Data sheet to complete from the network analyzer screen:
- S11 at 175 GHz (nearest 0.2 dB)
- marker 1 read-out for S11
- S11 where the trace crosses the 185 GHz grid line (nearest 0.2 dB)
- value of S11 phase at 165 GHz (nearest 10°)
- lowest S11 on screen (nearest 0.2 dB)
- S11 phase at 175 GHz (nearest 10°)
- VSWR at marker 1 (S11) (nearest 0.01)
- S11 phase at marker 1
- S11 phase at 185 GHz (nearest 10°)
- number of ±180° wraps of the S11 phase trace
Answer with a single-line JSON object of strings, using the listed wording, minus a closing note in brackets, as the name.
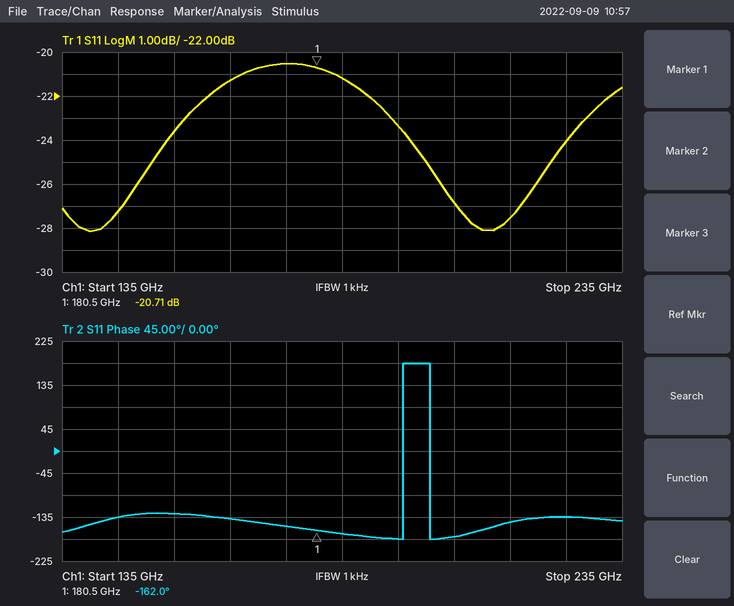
{"S11 at 175 GHz": "-20.6 dB", "marker 1 read-out for S11": "-20.71 dB", "S11 where the trace crosses the 185 GHz grid line": "-21.2 dB", "value of S11 phase at 165 GHz": "-140°", "lowest S11 on screen": "-28.2 dB", "S11 phase at 175 GHz": "-150°", "VSWR at marker 1 (S11)": "1.20", "S11 phase at marker 1": "-162.0°", "S11 phase at 185 GHz": "-170°", "number of ±180° wraps of the S11 phase trace": "2"}
